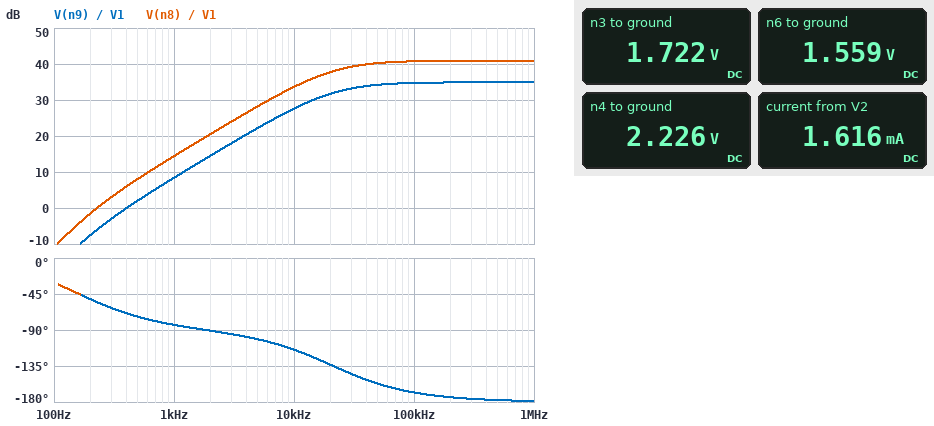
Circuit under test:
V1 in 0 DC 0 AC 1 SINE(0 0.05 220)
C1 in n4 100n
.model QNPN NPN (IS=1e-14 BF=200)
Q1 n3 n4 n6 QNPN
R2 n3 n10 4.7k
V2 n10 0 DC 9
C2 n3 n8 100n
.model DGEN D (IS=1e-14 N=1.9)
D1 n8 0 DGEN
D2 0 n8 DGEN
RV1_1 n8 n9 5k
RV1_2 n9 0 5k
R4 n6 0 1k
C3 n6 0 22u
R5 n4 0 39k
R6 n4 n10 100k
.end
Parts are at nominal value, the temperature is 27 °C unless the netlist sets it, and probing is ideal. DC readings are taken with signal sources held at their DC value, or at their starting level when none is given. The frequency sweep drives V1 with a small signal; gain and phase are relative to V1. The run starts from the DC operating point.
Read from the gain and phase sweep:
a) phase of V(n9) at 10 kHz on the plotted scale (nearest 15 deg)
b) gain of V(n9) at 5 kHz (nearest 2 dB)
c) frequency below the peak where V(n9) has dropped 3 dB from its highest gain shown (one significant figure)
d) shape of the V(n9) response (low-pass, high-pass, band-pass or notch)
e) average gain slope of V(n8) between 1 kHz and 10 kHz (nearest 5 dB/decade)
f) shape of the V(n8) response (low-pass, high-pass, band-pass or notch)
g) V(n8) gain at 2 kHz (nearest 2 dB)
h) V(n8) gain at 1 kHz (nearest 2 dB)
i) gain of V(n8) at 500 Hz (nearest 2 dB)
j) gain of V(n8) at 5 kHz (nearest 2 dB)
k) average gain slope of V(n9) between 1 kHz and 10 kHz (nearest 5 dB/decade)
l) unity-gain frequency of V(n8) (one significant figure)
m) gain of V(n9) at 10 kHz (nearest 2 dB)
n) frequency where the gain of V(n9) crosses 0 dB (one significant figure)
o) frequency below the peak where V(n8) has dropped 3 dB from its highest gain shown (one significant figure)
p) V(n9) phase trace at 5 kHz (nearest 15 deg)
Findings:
-120 deg
22 dB
20 kHz
high-pass
20 dB/decade
high-pass
20 dB
14 dB
8 dB
28 dB
20 dB/decade
200 Hz
28 dB
400 Hz
20 kHz
-105 deg
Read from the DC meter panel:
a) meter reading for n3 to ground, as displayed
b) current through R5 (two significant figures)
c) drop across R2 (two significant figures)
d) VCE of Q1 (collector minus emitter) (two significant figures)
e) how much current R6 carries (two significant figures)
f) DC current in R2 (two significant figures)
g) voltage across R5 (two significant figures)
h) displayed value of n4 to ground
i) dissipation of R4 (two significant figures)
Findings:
1.722 V
57 µA
7.3 V
160 mV
68 µA
1.5 mA
2.2 V
2.226 V
2.4 mW
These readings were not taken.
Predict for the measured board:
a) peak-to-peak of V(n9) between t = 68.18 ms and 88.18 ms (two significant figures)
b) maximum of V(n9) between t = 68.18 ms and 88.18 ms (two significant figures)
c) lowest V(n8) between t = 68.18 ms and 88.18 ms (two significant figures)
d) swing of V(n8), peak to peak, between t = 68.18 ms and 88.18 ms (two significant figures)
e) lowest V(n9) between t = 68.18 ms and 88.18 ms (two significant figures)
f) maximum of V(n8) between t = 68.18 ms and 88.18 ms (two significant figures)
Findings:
560 mV
320 mV
-480 mV
1.1 V
-240 mV
640 mV
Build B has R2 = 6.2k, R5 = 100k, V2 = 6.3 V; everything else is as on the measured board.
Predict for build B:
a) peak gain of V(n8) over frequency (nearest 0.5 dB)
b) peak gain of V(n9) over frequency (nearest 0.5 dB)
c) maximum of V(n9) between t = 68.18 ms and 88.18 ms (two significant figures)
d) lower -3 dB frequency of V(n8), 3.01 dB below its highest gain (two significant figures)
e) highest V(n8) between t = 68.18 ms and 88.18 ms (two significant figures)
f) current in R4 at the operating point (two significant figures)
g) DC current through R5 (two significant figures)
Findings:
23.0 dB
17.0 dB
2.6 mV
26 kHz
5.1 mV
890 µA
15 µA
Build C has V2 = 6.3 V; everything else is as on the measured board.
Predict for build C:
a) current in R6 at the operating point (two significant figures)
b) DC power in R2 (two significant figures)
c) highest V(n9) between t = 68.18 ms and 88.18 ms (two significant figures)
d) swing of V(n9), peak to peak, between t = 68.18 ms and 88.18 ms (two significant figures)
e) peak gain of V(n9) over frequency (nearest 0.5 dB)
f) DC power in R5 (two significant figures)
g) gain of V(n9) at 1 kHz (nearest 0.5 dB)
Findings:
47 µA
4.4 mW
530 mV
1.1 V
35.5 dB
68 µW
34.0 dB
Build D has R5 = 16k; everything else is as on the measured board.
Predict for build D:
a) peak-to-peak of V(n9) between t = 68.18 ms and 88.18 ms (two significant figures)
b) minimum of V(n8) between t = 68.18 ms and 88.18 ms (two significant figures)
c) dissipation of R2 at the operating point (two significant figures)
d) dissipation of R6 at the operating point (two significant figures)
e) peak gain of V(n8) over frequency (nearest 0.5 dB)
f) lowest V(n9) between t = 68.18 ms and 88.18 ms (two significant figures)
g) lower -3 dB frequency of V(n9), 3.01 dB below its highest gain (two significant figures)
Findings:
1.1 V
-1.1 V
1.5 mW
610 µW
37.0 dB
-570 mV
430 Hz
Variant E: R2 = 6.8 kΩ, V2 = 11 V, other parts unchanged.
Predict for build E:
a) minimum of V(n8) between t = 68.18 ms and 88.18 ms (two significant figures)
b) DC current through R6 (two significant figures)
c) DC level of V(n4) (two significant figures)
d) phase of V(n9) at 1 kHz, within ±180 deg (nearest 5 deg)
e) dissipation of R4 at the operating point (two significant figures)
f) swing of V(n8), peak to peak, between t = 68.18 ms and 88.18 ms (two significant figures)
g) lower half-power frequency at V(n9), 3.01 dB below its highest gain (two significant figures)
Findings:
-4.7 mV
89 µA
2.1 V
-80 deg
2.0 mW
9.9 mV
41 kHz
